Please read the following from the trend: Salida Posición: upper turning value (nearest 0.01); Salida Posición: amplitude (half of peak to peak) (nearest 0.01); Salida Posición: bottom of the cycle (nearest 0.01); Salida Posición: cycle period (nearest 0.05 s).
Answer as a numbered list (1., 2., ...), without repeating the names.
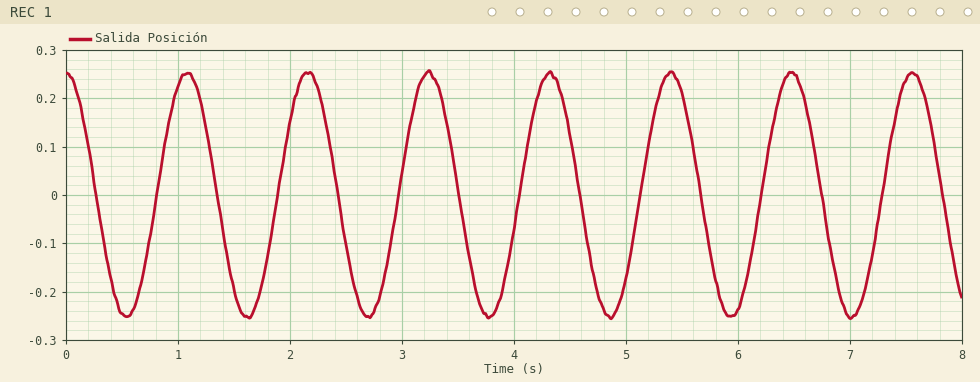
1. 0.25
2. 0.25
3. -0.25
4. 1.10 s
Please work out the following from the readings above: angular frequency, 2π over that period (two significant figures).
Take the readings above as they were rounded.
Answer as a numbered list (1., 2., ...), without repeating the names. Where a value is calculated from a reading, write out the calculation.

1. 2π / 1.1 = 5.7 rad/s
